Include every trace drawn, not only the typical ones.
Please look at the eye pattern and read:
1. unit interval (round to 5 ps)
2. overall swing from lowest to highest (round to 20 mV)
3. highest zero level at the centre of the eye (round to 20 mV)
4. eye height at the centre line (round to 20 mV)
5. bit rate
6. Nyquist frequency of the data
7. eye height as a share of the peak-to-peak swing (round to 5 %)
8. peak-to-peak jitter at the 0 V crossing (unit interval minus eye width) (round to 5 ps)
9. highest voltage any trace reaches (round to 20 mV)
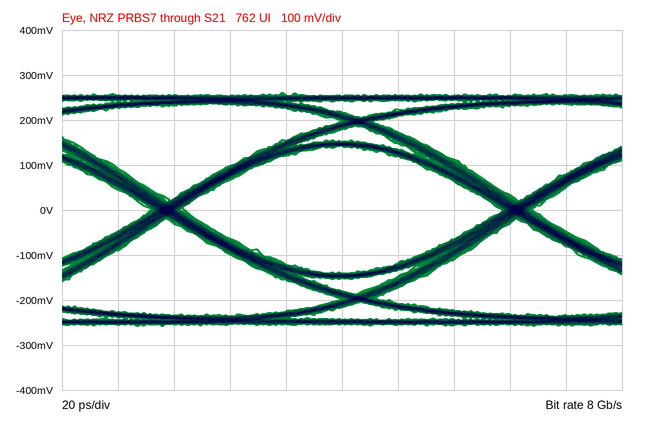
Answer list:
125 ps
520 mV
-140 mV
280 mV
8 Gb/s
4 GHz
55 %
10 ps
260 mV
